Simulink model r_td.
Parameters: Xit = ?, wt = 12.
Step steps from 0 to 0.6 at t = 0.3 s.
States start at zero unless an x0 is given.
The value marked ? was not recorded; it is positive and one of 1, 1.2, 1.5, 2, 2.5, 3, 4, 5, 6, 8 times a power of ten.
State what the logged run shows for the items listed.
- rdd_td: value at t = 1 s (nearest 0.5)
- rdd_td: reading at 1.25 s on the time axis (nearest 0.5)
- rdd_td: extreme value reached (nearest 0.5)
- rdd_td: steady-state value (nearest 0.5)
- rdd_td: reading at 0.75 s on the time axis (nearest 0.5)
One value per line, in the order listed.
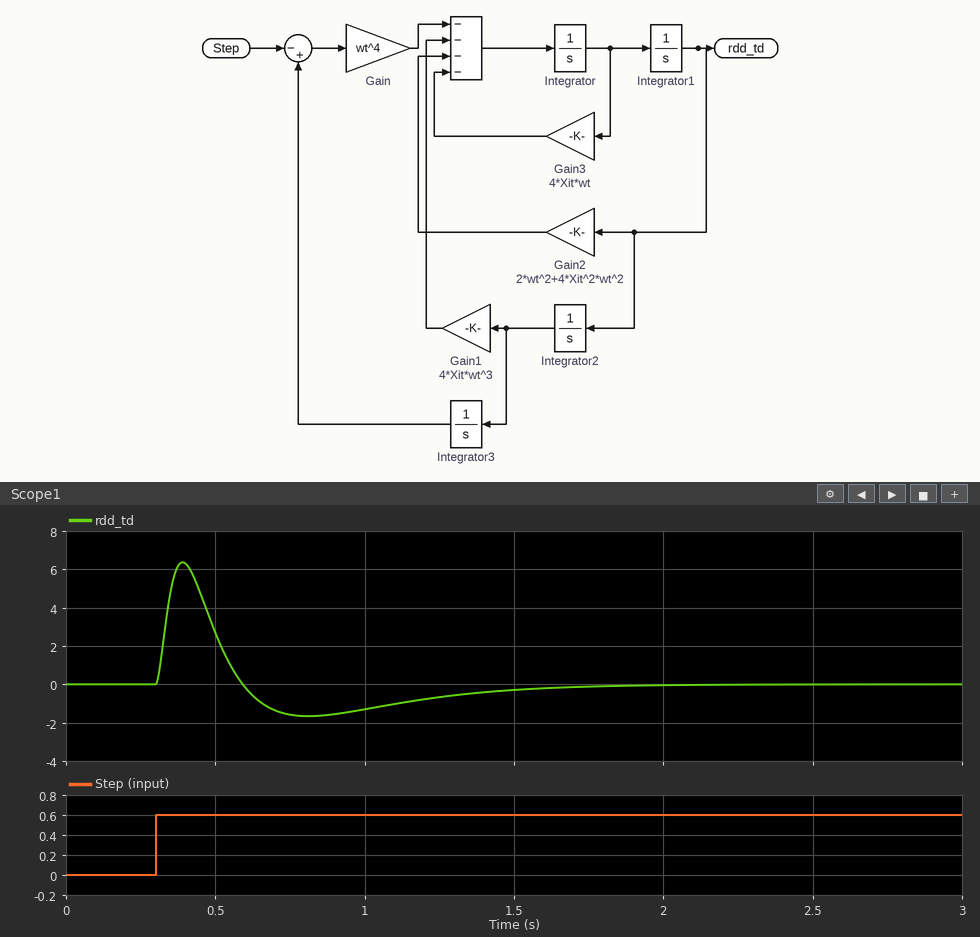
-1.5
-0.5
6.5
0.0
-1.5
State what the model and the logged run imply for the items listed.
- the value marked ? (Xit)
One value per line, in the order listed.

1.5
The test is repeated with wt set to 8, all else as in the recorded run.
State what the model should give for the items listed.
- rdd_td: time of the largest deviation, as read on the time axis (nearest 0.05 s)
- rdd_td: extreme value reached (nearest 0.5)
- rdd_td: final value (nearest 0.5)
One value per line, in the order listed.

0.45 s
3.0
0.0
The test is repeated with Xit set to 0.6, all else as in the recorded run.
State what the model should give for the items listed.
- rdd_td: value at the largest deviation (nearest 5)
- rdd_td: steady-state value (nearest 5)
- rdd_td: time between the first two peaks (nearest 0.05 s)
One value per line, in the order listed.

20
0
0.55 s
